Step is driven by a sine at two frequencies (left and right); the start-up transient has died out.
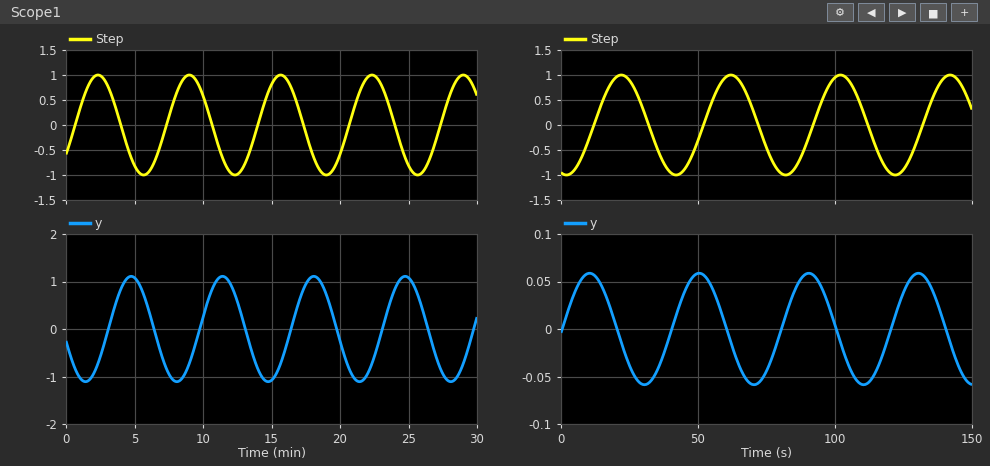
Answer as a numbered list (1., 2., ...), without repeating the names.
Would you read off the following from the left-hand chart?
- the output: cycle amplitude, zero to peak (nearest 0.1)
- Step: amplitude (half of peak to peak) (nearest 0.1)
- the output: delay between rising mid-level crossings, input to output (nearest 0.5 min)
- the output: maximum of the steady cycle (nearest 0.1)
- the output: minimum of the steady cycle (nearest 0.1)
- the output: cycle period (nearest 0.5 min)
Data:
1. 1.1
2. 1.0
3. 2.5 min
4. 1.1
5. -1.1
6. 6.5 min
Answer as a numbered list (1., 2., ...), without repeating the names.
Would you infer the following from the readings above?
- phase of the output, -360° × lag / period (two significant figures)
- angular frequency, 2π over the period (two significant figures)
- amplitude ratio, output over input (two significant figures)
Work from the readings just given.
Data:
1. -140°
2. 0.97 rad/min
3. 1.1
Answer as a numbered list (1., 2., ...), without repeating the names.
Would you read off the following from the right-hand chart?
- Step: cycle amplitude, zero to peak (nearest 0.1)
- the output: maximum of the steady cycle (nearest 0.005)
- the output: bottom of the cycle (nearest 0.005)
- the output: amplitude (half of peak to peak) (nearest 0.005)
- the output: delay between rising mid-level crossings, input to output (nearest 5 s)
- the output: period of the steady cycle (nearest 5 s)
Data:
1. 1.0
2. 0.060
3. -0.060
4. 0.060
5. 30 s
6. 40 s
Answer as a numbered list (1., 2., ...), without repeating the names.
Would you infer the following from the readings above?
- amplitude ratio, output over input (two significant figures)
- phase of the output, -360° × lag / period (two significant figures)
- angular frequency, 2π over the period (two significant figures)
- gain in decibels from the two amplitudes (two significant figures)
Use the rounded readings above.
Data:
1. 0.060
2. -270°
3. 0.16 rad/s
4. -24 dB
